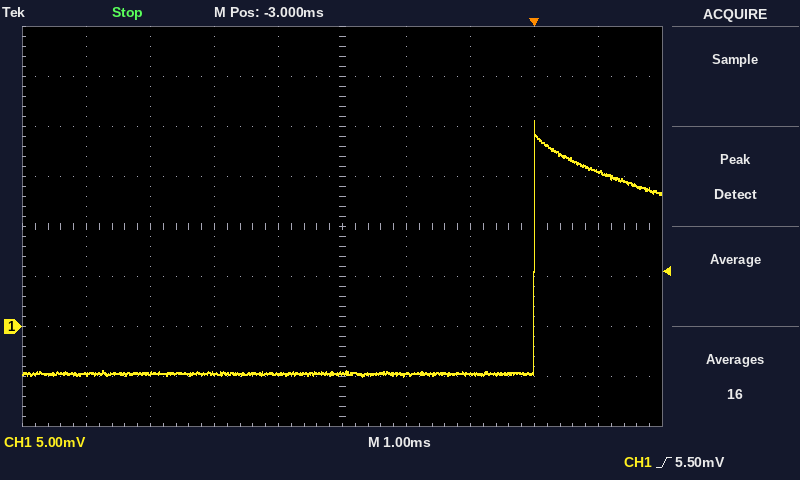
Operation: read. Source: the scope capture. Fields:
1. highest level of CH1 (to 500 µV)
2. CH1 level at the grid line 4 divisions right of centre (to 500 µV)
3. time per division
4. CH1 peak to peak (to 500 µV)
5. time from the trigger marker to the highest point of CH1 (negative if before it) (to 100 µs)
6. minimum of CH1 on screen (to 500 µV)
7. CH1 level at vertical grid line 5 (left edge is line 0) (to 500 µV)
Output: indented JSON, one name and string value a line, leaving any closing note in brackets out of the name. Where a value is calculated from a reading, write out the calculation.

{
  "highest level of CH1": "20.5 mV",
  "CH1 level at the grid line 4 divisions right of centre": "15.5 mV",
  "time per division": "1 ms",
  "CH1 peak to peak": "20.5 mV − (-5.0 mV) = 25.5 mV",
  "time from the trigger marker to the highest point of CH1 (negative if before it)": "0.0 ms",
  "minimum of CH1 on screen": "-5.0 mV",
  "CH1 level at vertical grid line 5 (left edge is line 0)": "-4.5 mV"
}
